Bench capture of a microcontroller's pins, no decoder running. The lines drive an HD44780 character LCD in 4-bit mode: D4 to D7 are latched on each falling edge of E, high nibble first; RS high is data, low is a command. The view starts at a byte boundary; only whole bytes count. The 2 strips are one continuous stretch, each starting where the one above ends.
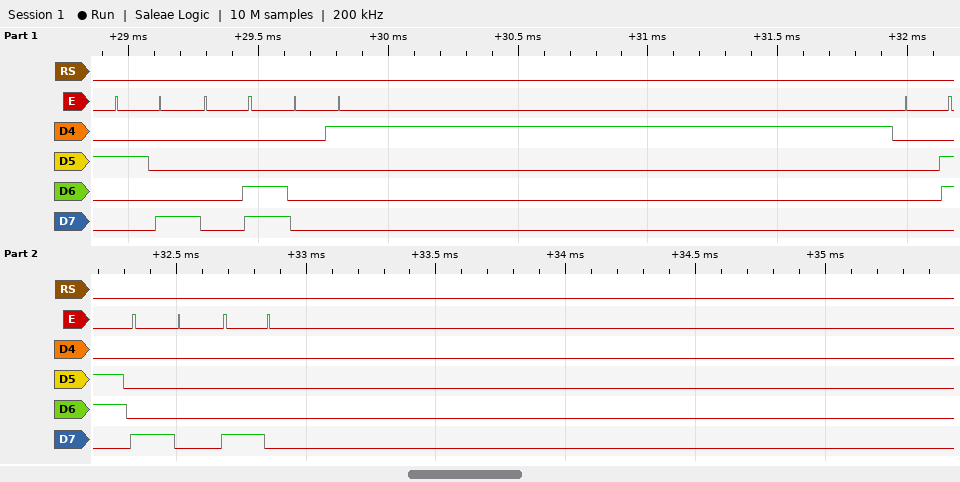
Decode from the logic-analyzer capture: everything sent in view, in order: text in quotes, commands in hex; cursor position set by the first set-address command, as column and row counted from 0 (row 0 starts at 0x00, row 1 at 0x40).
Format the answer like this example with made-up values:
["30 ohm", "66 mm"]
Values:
["0x28 0x0C 0x01 0x06 0x80 0x80", "column 0, row 0"]
